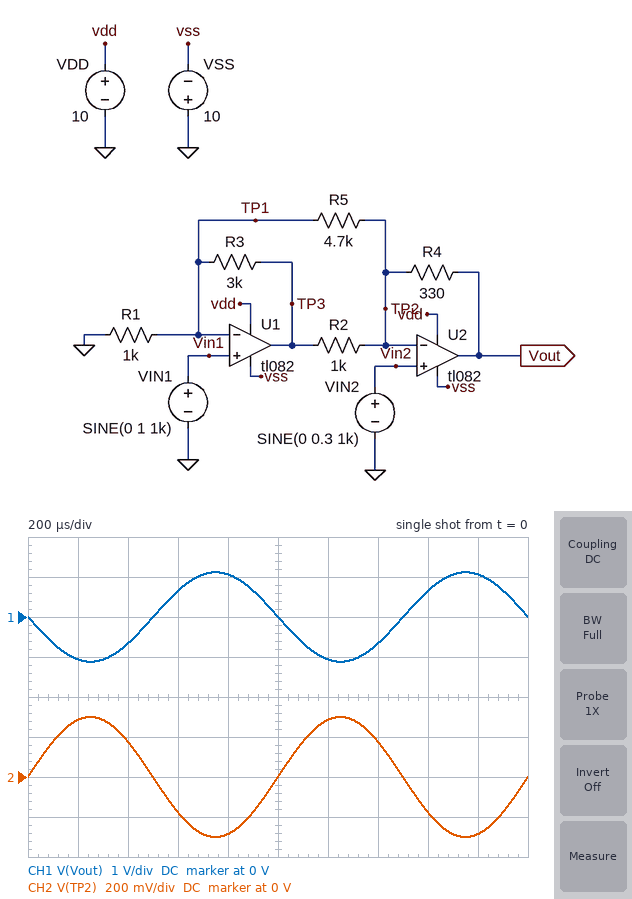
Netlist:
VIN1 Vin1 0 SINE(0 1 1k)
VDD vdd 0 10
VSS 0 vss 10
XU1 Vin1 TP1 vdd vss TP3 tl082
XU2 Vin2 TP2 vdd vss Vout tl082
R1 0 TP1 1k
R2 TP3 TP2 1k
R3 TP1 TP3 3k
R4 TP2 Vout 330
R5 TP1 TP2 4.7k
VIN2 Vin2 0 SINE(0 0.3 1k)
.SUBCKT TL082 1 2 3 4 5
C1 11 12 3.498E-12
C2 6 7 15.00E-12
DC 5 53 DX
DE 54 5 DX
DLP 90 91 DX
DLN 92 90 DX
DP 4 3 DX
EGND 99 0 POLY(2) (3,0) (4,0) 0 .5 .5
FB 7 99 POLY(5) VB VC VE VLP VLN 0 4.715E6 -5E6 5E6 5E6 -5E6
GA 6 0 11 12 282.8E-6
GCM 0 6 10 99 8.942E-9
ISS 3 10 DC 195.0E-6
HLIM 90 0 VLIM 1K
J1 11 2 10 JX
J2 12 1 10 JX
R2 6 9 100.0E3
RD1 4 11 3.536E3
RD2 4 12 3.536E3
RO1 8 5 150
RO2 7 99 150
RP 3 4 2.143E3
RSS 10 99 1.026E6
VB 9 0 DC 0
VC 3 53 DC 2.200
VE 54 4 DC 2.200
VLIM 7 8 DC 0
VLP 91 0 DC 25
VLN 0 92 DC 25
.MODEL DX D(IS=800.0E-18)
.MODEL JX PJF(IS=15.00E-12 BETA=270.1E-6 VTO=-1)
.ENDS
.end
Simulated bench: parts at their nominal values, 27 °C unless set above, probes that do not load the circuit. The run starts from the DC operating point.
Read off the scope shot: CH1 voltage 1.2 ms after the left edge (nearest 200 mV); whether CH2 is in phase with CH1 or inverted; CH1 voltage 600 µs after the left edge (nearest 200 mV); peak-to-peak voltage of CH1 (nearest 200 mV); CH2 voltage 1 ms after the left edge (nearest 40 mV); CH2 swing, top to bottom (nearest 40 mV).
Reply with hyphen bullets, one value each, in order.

- -1.0 V
- inverted
- 600 mV
- 2.2 V
- 0 V
- 600 mV
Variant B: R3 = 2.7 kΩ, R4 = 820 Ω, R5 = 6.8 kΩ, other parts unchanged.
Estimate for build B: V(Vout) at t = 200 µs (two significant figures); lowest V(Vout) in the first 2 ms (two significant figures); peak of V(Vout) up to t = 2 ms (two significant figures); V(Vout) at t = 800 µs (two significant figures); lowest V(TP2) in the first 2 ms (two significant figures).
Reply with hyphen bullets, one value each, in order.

- -2.7 V
- -2.8 V
- 2.8 V
- 2.7 V
- -300 mV
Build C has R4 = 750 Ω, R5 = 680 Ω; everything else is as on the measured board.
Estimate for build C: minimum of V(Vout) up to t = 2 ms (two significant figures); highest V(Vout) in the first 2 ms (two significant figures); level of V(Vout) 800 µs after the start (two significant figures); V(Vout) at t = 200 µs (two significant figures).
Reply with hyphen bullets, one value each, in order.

- -5.6 V
- 5.6 V
- 5.3 V
- -5.3 V
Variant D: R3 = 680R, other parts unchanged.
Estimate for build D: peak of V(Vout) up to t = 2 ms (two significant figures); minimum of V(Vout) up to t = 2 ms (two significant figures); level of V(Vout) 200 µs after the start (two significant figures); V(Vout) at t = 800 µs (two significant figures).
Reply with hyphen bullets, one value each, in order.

- 240 mV
- -240 mV
- -230 mV
- 230 mV
